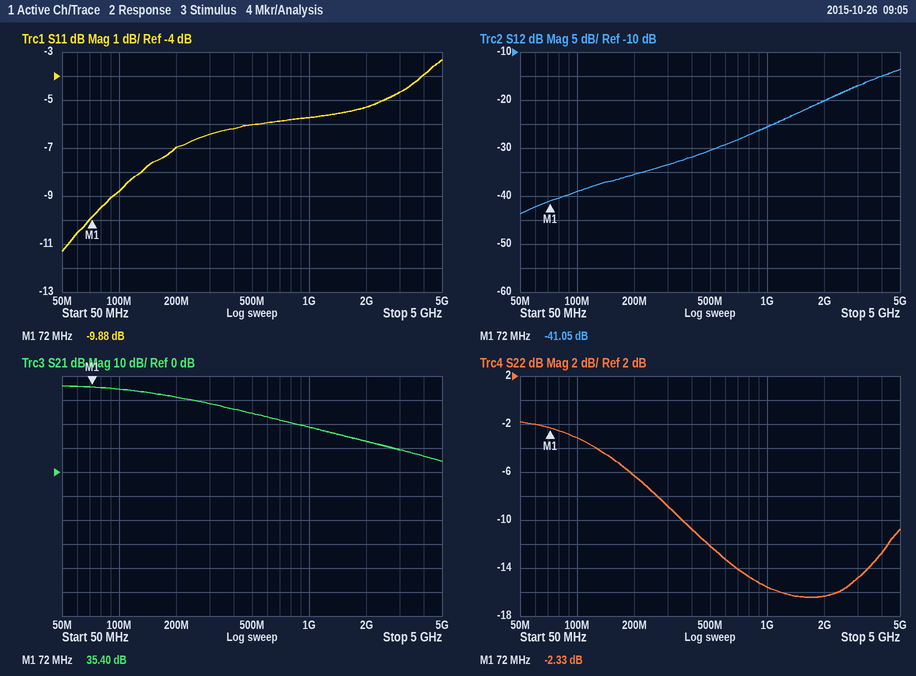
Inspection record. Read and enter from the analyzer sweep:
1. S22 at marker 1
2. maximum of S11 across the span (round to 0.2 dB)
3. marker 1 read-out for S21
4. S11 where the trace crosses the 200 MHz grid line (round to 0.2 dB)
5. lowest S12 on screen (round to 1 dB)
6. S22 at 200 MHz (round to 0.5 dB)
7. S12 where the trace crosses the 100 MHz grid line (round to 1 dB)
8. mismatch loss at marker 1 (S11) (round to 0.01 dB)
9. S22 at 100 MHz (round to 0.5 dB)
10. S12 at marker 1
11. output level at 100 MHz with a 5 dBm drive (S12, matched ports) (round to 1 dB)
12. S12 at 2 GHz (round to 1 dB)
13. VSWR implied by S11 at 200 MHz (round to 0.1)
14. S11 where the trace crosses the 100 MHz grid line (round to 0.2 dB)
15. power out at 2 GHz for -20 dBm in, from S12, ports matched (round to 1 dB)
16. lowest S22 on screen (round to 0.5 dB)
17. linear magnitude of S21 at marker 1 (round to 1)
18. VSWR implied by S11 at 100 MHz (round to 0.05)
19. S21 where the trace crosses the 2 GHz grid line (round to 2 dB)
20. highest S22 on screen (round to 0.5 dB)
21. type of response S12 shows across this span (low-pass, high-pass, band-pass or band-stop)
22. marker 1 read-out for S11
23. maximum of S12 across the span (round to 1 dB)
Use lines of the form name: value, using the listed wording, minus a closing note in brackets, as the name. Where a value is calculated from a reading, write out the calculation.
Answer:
S22 at marker 1: -2.33 dB
maximum of S11 across the span: -3.4 dB
marker 1 read-out for S21: 35.40 dB
S11 where the trace crosses the 200 MHz grid line: -7.0 dB
lowest S12 on screen: -44 dB
S22 at 200 MHz: -6.5 dB
S12 where the trace crosses the 100 MHz grid line: -39 dB
mismatch loss at marker 1 (S11): −10 log10(1 − 10^(-9.88/10)) ≈ 0.47 dB
S22 at 100 MHz: -3.0 dB
S12 at marker 1: -41.05 dB
output level at 100 MHz with a 5 dBm drive (S12, matched ports): 5 dBm + (-39 dB) = -34 dBm
S12 at 2 GHz: -20 dB
VSWR implied by S11 at 200 MHz: |Γ| = 10^(-7/20) = 0.4467; VSWR = (1 + 0.4467)/(1 − 0.4467) ≈ 2.6
S11 where the trace crosses the 100 MHz grid line: -8.8 dB
power out at 2 GHz for -20 dBm in, from S12, ports matched: -20 dBm + (-20 dB) = -40 dBm
lowest S22 on screen: -16.5 dB
linear magnitude of S21 at marker 1: 10^(35.4/20) ≈ 59
VSWR implied by S11 at 100 MHz: |Γ| = 10^(-8.8/20) = 0.3631; VSWR = (1 + 0.3631)/(1 − 0.3631) ≈ 2.14, so 2.15 to the nearest 0.05
S21 where the trace crosses the 2 GHz grid line: 12 dB
highest S22 on screen: -2.0 dB
type of response S12 shows across this span: high-pass
marker 1 read-out for S11: -9.88 dB
maximum of S12 across the span: -14 dB
